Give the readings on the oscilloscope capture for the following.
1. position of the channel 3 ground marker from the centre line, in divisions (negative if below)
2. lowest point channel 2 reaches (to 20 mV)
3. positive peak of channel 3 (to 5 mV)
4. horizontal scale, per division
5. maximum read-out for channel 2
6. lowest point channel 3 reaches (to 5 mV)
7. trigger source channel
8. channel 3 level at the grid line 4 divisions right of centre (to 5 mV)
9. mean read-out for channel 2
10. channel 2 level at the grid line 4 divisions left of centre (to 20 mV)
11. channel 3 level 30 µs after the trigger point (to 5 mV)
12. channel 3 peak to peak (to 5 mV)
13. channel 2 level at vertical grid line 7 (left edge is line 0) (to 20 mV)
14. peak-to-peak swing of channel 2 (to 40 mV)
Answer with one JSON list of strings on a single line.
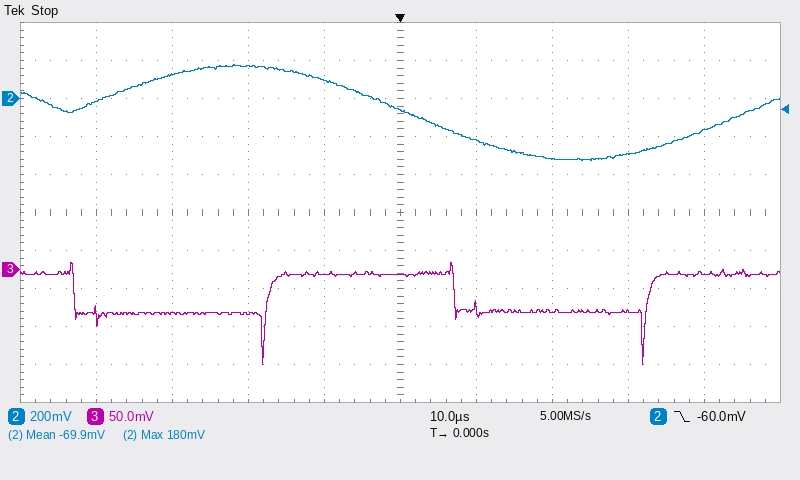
["-1.5 div", "-320 mV", "10 mV", "10 µs", "180 mV", "-125 mV", "channel 2", "-5 mV", "-69.9 mV", "-20 mV", "-55 mV", "135 mV", "-320 mV", "520 mV"]
